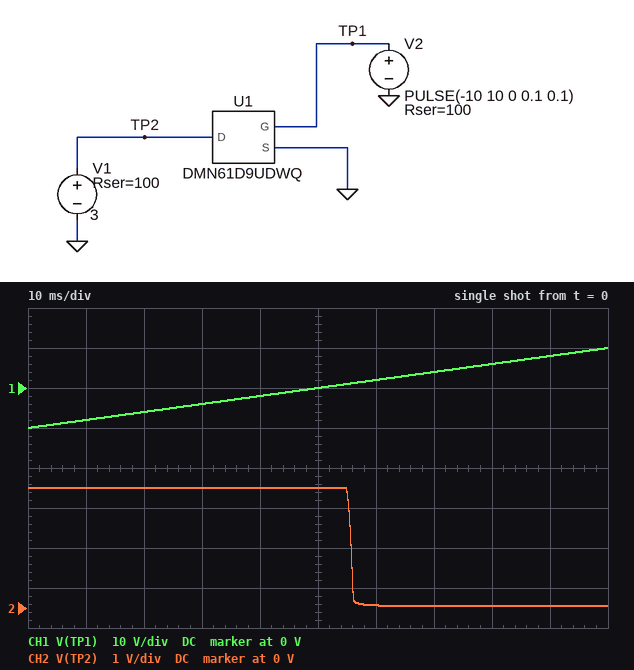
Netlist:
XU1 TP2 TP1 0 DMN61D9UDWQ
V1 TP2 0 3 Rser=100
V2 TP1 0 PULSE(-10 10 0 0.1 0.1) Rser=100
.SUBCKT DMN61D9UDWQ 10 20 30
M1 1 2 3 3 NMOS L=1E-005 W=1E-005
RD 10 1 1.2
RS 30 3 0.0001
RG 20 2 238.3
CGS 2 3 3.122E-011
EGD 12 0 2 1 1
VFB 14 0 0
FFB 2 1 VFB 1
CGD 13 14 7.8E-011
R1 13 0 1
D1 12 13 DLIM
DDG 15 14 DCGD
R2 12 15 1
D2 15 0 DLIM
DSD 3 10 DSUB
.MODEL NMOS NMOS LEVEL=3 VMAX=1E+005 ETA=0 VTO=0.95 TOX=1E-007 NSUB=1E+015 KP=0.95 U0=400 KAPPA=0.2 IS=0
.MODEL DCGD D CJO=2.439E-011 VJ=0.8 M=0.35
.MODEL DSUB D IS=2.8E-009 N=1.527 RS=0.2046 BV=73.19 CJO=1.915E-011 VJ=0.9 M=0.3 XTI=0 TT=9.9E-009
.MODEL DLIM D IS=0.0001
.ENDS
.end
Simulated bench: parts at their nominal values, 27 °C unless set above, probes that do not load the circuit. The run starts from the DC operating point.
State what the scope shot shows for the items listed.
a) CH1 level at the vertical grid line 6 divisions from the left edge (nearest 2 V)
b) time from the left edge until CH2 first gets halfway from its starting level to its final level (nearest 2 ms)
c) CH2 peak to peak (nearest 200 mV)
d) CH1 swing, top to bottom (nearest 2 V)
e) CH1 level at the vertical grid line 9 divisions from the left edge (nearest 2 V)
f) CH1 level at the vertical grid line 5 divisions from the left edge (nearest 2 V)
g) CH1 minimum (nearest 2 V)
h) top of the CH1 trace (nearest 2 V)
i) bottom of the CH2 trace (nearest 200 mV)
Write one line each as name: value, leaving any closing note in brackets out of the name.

CH1 level at the vertical grid line 6 divisions from the left edge: 2 V
time from the left edge until CH2 first gets halfway from its starting level to its final level: 56 ms
CH2 peak to peak: 3.0 V
CH1 swing, top to bottom: 20 V
CH1 level at the vertical grid line 9 divisions from the left edge: 8 V
CH1 level at the vertical grid line 5 divisions from the left edge: 0 V
CH1 minimum: -10 V
top of the CH1 trace: 10 V
bottom of the CH2 trace: 0 V
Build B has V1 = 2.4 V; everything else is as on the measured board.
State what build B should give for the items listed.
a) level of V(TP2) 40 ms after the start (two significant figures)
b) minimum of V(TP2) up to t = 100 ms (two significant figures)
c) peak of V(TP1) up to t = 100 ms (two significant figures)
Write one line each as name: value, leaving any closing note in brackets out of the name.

level of V(TP2) 40 ms after the start: 2.4 V
minimum of V(TP2) up to t = 100 ms: 31 mV
peak of V(TP1) up to t = 100 ms: 10 V
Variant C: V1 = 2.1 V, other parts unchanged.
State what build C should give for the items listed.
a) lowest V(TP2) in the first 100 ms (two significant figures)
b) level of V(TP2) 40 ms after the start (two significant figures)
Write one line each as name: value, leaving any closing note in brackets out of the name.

lowest V(TP2) in the first 100 ms: 27 mV
level of V(TP2) 40 ms after the start: 2.1 V
